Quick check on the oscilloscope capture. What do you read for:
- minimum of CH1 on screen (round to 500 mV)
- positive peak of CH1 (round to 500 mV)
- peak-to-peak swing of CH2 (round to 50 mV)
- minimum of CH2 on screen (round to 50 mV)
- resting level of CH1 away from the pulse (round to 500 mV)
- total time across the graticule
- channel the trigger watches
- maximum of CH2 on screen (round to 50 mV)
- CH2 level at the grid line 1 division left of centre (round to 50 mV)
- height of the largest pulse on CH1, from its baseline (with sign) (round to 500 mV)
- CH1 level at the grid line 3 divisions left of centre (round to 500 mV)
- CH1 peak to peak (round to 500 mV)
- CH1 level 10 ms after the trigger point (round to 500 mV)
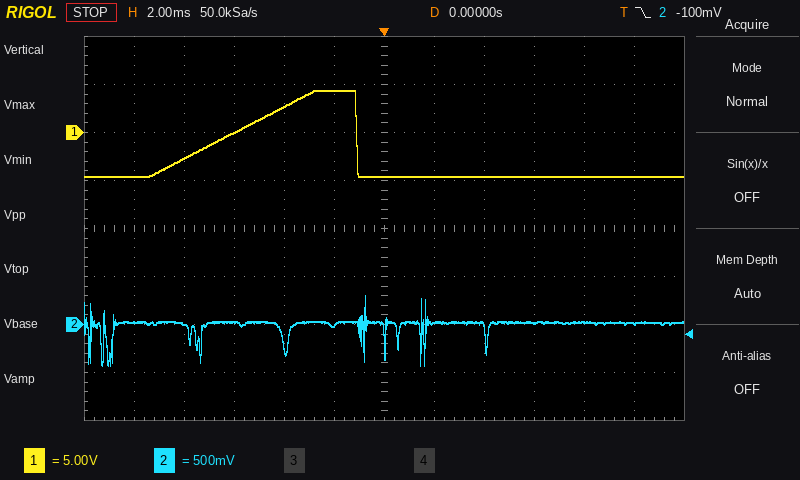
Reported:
-4.5 V
4.5 V
750 mV
-450 mV
-4.5 V
24 ms
CH2
300 mV
0 mV
+9.0 V
0.0 V
9.0 V
-4.5 V
